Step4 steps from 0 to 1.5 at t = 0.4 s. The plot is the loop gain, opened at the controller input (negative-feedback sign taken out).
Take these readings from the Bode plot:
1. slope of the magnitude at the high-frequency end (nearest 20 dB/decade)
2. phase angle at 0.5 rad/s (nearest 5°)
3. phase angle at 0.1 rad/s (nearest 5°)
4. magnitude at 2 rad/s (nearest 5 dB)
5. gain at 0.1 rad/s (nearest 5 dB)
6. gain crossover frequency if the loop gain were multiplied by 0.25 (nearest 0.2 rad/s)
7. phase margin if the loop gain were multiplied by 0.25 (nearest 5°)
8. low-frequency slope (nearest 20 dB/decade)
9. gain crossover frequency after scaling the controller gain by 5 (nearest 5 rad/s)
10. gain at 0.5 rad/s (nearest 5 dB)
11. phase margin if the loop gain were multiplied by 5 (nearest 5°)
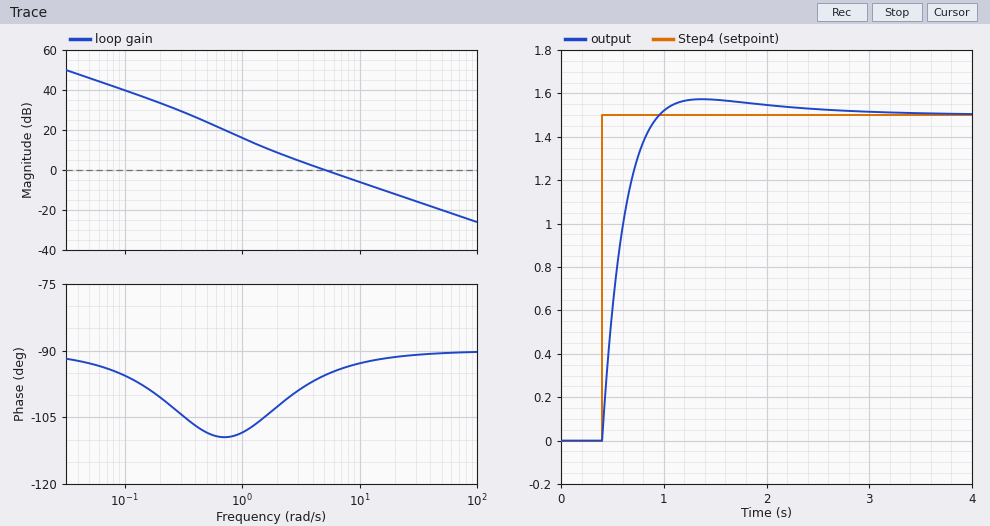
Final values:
-20 dB/decade
-110°
-95°
10 dB
40 dB
1.4 rad/s
75°
-20 dB/decade
25 rad/s
25 dB
90°
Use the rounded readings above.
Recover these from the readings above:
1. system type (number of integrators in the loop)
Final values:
1
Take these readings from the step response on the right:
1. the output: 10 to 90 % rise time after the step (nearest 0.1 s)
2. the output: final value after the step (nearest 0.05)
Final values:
0.4 s
1.50
